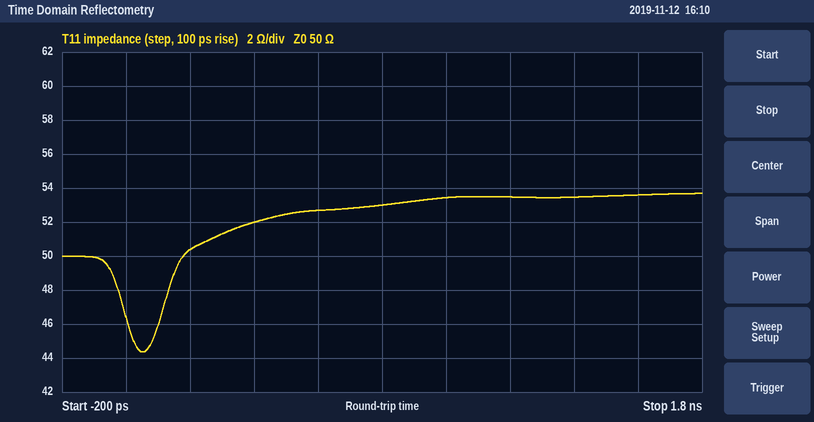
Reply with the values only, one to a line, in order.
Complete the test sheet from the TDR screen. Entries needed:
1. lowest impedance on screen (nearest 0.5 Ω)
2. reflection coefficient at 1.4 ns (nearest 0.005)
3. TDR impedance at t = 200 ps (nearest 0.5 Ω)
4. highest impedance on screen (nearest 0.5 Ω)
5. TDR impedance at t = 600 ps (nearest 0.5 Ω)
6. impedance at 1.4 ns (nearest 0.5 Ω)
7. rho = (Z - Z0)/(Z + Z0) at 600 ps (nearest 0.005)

44.5 Ω
+0.035
50.5 Ω
53.5 Ω
52.5 Ω
53.5 Ω
+0.025
